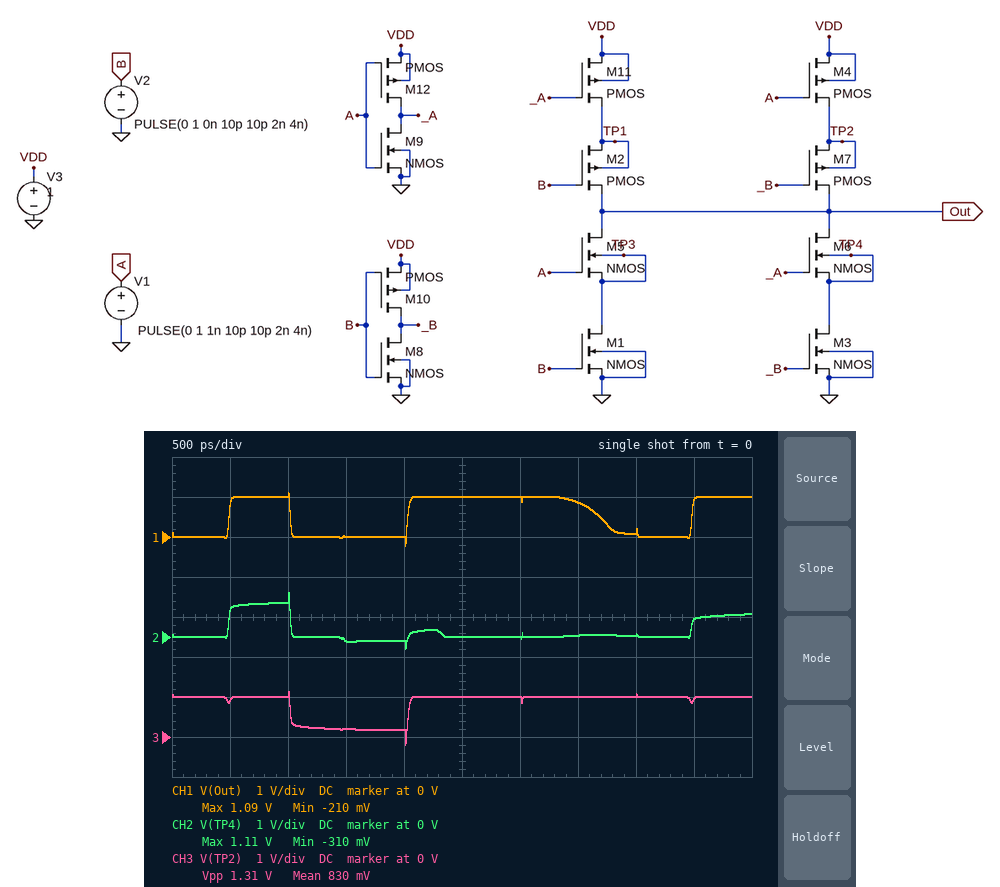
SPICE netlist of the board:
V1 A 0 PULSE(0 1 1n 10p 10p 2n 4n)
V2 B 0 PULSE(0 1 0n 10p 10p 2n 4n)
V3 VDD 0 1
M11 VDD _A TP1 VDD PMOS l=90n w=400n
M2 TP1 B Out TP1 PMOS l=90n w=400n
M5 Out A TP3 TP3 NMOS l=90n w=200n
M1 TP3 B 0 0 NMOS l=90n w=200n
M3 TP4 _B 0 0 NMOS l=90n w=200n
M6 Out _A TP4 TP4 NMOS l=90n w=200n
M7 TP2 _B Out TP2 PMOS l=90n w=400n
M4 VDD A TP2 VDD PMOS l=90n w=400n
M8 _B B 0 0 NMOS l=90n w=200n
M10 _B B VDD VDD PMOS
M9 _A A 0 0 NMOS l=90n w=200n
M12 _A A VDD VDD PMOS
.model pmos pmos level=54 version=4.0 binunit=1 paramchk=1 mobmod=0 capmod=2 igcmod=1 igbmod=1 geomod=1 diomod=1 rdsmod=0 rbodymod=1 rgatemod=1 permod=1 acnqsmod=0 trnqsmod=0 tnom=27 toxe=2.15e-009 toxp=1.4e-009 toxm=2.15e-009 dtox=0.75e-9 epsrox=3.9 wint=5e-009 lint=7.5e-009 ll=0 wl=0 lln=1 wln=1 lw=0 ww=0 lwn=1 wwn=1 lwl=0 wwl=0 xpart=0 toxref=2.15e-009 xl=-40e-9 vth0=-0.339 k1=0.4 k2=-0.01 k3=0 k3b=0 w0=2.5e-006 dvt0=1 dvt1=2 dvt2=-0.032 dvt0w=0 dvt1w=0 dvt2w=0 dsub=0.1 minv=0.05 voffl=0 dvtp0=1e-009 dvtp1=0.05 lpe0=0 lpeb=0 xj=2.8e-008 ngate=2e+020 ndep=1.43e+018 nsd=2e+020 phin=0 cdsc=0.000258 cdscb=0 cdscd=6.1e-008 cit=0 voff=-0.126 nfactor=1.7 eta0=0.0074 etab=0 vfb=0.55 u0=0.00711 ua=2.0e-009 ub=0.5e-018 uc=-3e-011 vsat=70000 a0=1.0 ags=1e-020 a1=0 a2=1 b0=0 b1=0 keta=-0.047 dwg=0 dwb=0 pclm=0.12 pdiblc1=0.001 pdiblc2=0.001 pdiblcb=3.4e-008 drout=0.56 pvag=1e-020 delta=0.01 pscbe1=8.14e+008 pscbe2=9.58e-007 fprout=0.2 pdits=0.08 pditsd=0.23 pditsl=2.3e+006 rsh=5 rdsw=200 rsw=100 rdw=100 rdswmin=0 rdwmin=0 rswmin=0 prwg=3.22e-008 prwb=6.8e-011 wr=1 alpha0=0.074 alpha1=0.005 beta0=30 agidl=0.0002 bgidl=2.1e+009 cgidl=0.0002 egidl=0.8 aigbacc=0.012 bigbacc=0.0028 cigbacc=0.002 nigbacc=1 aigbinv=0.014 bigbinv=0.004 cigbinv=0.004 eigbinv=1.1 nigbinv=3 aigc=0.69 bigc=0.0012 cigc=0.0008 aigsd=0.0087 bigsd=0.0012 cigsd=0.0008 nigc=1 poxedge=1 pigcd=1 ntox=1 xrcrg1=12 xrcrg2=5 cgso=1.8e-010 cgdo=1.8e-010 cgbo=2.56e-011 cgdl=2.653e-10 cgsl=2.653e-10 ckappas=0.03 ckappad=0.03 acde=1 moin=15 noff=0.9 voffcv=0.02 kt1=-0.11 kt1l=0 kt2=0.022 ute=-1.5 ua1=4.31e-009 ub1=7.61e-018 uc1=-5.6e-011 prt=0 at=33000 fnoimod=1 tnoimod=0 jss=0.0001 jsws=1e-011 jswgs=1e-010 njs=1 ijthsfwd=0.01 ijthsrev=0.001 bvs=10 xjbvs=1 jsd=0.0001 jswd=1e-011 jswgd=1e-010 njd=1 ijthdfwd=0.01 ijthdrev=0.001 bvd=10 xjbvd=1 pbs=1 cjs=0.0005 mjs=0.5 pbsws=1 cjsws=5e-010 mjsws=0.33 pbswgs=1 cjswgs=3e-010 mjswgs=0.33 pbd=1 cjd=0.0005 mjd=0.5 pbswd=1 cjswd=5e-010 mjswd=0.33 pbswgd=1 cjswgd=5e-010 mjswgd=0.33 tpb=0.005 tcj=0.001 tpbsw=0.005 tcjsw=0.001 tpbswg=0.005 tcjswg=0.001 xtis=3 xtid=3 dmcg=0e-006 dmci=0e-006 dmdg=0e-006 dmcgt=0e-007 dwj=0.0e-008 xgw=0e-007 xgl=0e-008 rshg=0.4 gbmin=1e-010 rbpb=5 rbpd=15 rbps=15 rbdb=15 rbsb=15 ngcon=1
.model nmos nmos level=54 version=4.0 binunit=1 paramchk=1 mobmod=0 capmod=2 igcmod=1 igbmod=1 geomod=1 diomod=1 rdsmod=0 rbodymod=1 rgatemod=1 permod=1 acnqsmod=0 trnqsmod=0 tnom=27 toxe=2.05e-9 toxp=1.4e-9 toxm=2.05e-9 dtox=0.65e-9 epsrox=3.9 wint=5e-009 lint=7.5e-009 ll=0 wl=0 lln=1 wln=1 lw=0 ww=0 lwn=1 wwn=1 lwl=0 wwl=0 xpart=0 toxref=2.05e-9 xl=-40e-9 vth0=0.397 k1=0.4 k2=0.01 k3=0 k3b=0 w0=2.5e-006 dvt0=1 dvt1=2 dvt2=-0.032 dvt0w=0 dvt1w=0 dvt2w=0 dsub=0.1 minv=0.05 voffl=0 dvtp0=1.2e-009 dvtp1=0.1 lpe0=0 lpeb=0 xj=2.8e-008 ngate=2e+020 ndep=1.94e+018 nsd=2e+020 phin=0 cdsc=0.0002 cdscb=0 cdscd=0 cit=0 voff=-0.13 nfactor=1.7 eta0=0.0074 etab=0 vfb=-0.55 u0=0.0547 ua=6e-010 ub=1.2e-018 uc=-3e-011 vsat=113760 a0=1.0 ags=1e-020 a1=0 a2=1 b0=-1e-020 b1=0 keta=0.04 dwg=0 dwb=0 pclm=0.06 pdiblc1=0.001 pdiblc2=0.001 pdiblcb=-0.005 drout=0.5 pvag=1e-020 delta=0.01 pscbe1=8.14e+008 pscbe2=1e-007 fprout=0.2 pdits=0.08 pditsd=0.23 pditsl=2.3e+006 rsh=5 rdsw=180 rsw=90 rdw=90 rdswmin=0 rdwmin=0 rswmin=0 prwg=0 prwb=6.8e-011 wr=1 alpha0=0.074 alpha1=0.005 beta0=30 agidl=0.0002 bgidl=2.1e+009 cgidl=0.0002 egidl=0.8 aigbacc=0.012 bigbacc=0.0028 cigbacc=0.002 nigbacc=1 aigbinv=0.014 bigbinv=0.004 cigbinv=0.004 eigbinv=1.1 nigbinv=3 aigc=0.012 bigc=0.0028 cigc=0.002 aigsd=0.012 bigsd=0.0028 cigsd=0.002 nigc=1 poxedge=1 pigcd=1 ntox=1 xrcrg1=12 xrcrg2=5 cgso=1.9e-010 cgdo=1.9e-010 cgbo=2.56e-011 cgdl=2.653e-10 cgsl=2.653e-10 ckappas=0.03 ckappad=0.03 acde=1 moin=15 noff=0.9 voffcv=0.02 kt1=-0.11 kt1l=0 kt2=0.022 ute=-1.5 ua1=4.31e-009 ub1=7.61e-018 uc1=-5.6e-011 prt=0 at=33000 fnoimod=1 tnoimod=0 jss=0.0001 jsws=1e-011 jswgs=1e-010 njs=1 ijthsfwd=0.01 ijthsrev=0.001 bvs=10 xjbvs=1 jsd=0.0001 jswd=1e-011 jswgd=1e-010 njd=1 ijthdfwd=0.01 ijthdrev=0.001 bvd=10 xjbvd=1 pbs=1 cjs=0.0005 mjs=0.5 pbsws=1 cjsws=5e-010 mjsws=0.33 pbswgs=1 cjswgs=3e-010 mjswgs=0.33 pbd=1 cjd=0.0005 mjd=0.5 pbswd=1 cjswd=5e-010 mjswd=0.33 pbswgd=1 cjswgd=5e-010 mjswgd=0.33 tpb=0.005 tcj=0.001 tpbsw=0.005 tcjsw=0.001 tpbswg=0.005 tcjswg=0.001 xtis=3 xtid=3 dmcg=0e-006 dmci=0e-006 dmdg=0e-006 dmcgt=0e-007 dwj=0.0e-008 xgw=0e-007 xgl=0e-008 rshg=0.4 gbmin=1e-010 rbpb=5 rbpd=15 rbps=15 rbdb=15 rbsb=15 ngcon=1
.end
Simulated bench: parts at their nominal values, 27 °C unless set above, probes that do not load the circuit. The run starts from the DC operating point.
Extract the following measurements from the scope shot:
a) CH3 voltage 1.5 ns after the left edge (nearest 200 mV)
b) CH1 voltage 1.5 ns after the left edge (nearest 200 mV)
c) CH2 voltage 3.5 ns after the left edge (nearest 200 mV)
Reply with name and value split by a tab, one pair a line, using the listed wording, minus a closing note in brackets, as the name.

CH3 voltage 1.5 ns after the left edge	200 mV
CH1 voltage 1.5 ns after the left edge	0 V
CH2 voltage 3.5 ns after the left edge	0 V
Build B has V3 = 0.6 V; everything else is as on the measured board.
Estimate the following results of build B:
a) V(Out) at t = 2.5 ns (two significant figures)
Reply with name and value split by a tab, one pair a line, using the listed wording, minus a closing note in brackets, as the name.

V(Out) at t = 2.5 ns	600 mV
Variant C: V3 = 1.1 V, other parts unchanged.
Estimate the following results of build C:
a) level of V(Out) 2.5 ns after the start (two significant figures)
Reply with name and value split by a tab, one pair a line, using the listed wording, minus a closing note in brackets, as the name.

level of V(Out) 2.5 ns after the start	1.1 V
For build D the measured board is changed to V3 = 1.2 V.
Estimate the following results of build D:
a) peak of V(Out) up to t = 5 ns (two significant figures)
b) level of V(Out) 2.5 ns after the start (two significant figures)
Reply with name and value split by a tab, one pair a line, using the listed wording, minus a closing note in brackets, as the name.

peak of V(Out) up to t = 5 ns	1.3 V
level of V(Out) 2.5 ns after the start	1.2 V
